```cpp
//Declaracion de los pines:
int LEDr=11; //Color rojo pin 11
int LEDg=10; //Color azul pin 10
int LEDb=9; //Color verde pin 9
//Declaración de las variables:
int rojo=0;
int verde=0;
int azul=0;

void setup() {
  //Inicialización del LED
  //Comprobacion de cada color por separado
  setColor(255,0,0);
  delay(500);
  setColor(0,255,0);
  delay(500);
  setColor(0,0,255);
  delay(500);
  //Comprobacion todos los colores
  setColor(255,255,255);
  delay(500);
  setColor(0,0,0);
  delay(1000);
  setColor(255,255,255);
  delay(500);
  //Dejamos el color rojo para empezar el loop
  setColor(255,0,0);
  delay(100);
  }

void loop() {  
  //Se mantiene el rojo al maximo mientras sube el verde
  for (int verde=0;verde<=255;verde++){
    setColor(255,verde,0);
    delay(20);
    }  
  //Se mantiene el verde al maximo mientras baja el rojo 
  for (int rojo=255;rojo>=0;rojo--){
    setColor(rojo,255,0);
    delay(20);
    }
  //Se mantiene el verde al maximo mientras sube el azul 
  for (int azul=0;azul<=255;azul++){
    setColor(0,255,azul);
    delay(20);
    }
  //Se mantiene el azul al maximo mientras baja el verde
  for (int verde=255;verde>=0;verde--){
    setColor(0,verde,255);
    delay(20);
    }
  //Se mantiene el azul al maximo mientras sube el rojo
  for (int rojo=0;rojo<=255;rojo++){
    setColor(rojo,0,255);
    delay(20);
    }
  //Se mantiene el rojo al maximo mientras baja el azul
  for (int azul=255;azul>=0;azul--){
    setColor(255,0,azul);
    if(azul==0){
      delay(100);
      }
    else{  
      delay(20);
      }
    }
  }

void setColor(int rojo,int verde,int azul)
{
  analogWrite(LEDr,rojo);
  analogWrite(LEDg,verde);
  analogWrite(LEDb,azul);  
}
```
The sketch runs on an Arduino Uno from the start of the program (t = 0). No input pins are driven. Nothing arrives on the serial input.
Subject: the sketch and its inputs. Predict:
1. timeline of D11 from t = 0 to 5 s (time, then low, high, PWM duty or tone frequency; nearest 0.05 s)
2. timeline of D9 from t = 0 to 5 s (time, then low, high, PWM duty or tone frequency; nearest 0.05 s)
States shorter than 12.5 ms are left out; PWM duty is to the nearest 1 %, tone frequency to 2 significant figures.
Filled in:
0 s high; 0.5 s low; 1.5 s high; 2 s low; 3 s high
0 s low; 1 s high; 2 s low; 3 s high; 3.5 s low
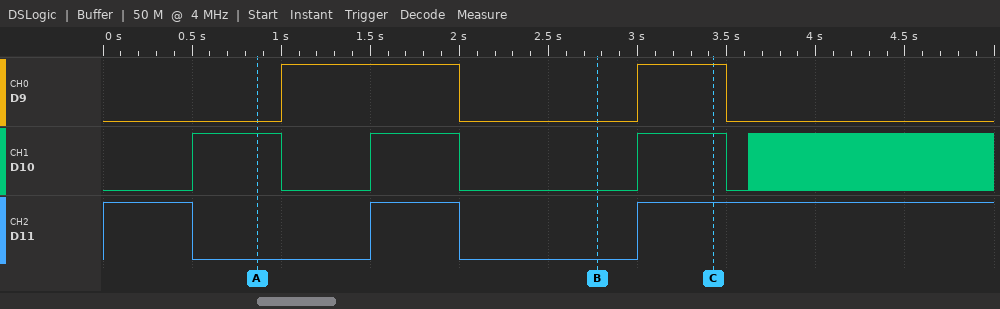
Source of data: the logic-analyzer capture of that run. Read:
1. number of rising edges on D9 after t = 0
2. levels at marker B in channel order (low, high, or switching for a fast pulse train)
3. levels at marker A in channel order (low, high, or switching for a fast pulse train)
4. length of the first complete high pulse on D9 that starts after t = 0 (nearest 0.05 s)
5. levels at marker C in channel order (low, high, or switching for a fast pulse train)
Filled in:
2
D9 low, D10 low, D11 low
D9 low, D10 high, D11 low
1.00 s
D9 high, D10 high, D11 high
